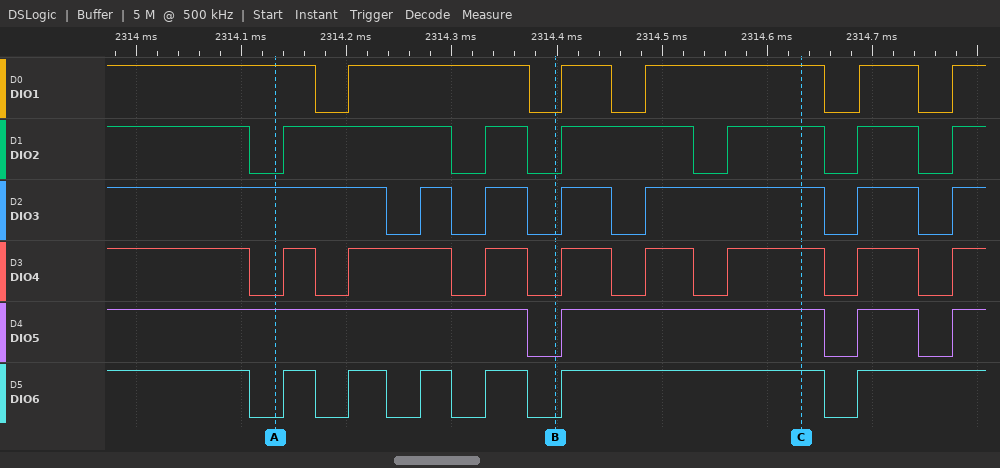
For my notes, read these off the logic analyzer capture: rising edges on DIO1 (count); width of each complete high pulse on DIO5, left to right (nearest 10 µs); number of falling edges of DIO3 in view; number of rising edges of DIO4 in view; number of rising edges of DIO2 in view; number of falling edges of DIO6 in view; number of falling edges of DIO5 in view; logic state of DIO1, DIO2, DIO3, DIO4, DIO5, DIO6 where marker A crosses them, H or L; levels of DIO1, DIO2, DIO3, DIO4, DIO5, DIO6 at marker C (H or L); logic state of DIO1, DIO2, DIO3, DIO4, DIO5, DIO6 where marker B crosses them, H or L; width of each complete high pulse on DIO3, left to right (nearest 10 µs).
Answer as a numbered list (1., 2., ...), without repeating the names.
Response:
1. 5
2. 250 µs, 60 µs
3. 6
4. 8
5. 6
6. 6
7. 3
8. DIO1=H, DIO2=L, DIO3=H, DIO4=L, DIO5=H, DIO6=L
9. DIO1=H, DIO2=H, DIO3=H, DIO4=H, DIO5=H, DIO6=H
10. DIO1=L, DIO2=L, DIO3=L, DIO4=L, DIO5=L, DIO6=L
11. 30 µs, 40 µs, 50 µs, 170 µs, 60 µs
